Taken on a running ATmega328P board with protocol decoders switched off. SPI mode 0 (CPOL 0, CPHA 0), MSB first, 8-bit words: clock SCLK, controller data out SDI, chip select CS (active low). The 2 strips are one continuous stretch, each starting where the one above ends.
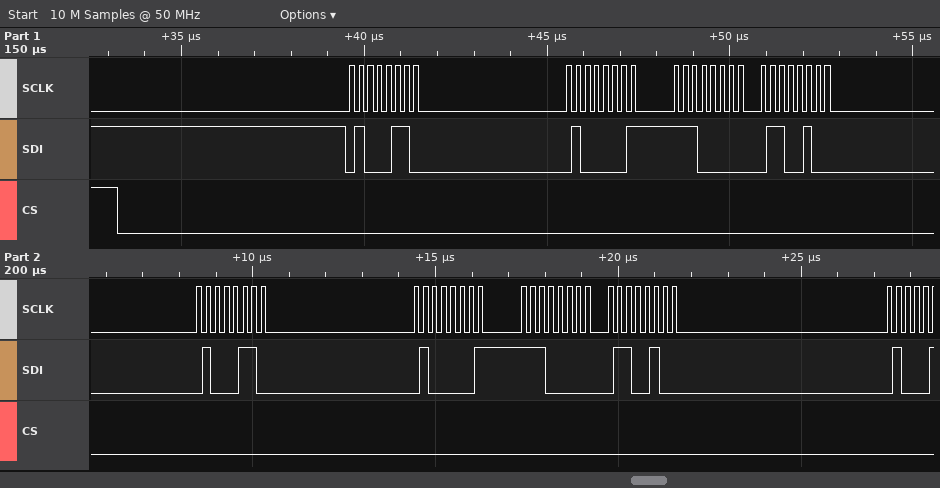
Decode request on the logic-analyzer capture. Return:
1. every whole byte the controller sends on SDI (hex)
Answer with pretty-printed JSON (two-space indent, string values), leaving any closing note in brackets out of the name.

{
  "every whole byte the controller sends on SDI": "0x46 0x41 0xE0 0x64 0x46 0x41 0xE0 0x64"
}
